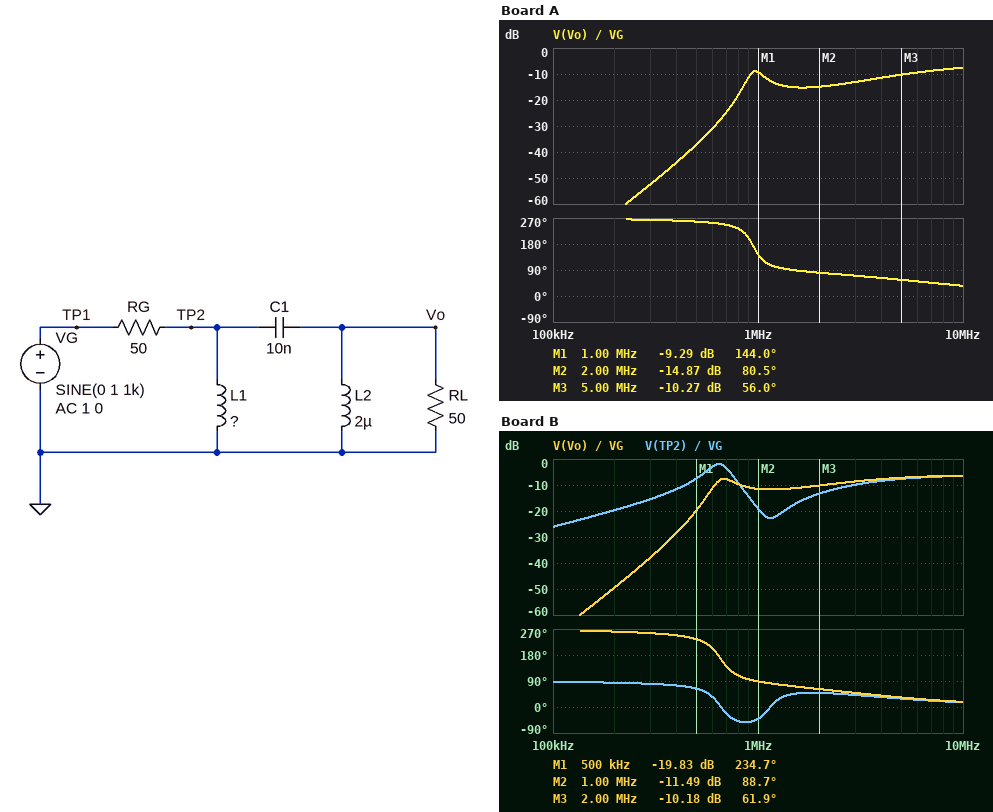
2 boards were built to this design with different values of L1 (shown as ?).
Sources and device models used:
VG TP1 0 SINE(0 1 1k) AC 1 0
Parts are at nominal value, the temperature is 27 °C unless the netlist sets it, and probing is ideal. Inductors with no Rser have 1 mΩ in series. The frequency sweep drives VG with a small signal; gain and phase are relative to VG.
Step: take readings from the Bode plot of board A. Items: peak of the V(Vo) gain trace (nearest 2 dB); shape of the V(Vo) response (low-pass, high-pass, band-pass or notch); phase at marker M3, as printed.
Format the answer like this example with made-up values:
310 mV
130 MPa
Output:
-8 dB
high-pass
56.0 deg
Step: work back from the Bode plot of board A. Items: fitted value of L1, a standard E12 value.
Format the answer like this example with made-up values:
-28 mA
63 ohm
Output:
820 nH
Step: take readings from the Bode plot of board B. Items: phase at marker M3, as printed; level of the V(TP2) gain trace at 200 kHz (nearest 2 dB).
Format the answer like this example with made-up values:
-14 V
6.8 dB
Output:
61.9 deg
-20 dB
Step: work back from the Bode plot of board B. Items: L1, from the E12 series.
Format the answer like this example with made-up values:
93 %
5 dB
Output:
3.9 µH
